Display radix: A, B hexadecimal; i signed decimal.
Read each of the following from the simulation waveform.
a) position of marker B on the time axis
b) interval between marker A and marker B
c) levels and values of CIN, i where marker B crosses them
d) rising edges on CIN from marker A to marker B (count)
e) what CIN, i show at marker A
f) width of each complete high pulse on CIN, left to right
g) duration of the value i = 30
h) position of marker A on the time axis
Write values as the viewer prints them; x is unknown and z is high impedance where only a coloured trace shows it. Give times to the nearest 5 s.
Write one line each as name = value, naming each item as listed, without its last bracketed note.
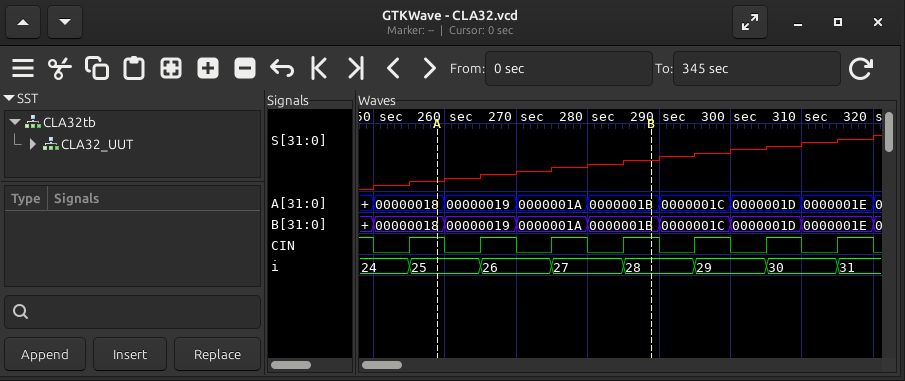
position of marker B on the time axis = 290 s
interval between marker A and marker B = 30 s
levels and values of CIN, i where marker B crosses them = CIN=1, i=28
rising edges on CIN from marker A to marker B = 3
what CIN, i show at marker A = CIN=1, i=25
width of each complete high pulse on CIN, left to right = 5 s, 5 s, 5 s, 5 s, 5 s, 5 s, 5 s
duration of the value i = 30 = 10 s
position of marker A on the time axis = 260 s
